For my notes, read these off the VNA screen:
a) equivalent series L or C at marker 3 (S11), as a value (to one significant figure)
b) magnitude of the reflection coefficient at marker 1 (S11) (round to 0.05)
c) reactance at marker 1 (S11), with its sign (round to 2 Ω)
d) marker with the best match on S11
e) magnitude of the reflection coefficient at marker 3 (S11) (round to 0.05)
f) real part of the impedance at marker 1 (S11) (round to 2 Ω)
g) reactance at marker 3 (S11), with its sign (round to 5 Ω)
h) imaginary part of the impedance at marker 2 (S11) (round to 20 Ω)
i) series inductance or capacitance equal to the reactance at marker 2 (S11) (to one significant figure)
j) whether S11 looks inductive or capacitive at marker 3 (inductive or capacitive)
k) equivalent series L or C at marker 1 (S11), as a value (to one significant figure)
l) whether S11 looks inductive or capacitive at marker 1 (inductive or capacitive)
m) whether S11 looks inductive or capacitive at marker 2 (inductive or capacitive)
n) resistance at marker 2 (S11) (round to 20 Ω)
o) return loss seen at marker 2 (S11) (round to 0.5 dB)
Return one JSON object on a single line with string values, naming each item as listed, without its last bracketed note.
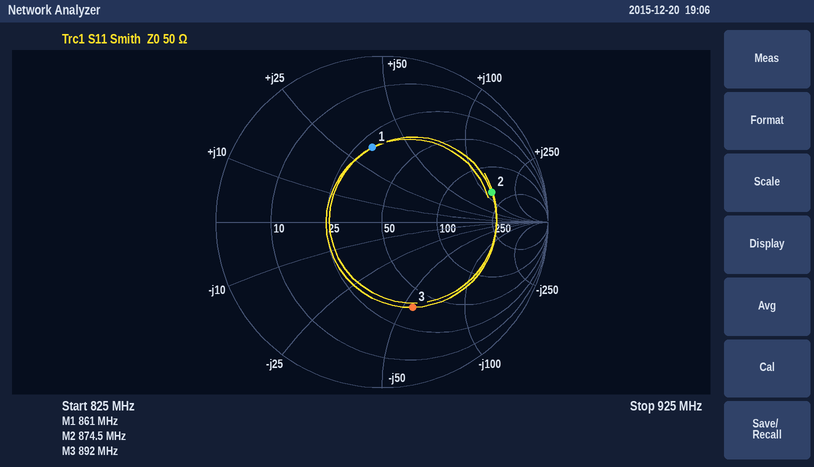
{"equivalent series L or C at marker 3 (S11), as a value": "3 pF", "magnitude of the reflection coefficient at marker 1 (S11)": "0.45", "reactance at marker 1 (S11), with its sign": "+34 Ω", "marker with the best match on S11": "marker 1", "magnitude of the reflection coefficient at marker 3 (S11)": "0.55", "real part of the impedance at marker 1 (S11)": "30 Ω", "reactance at marker 3 (S11), with its sign": "-55 Ω", "imaginary part of the impedance at marker 2 (S11)": "+120 Ω", "series inductance or capacitance equal to the reactance at marker 2 (S11)": "20 nH", "whether S11 looks inductive or capacitive at marker 3": "capacitive", "equivalent series L or C at marker 1 (S11), as a value": "6 nH", "whether S11 looks inductive or capacitive at marker 1": "inductive", "whether S11 looks inductive or capacitive at marker 2": "inductive", "resistance at marker 2 (S11)": "180 Ω", "return loss seen at marker 2 (S11)": "3.5 dB"}
